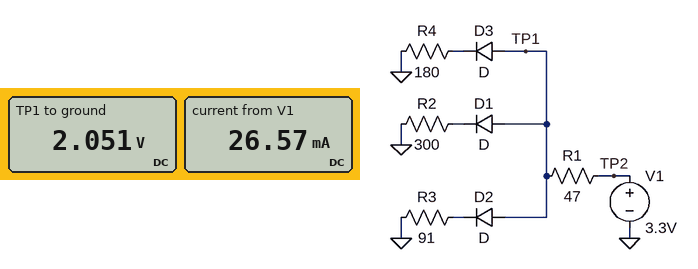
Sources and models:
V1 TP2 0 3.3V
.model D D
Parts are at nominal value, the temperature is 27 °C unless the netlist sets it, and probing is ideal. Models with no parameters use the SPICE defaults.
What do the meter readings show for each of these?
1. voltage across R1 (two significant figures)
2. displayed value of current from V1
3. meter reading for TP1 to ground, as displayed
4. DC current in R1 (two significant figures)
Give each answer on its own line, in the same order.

1.2 V
26.57 mA
2.051 V
27 mA
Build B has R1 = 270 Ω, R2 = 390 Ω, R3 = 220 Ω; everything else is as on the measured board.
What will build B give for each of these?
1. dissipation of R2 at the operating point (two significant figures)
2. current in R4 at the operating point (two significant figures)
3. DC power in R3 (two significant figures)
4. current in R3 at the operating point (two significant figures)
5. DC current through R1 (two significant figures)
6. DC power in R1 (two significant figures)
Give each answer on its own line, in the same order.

940 µW
3.3 mA
1.6 mW
2.7 mA
7.5 mA
15 mW
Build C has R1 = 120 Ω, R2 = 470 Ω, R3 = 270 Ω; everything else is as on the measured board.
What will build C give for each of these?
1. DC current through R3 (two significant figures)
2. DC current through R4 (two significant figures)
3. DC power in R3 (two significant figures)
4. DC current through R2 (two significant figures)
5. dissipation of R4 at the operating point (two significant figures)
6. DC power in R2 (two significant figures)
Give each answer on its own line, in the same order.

4.1 mA
6.1 mA
4.5 mW
2.4 mA
6.6 mW
2.7 mW
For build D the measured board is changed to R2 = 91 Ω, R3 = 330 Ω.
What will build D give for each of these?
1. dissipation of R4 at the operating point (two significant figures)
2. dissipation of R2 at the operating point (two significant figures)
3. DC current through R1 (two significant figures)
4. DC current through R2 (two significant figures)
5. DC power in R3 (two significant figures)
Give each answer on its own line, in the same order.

10 mW
20 mW
26 mA
15 mA
5.7 mW
